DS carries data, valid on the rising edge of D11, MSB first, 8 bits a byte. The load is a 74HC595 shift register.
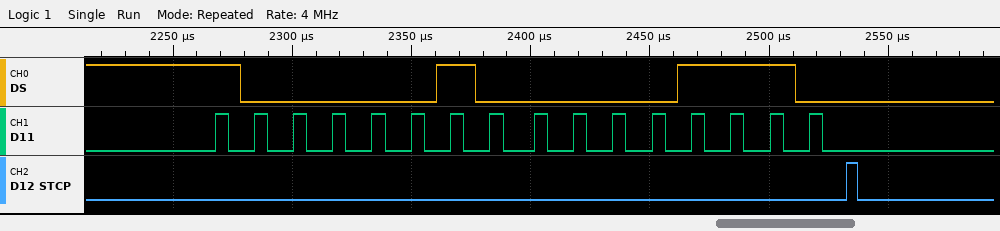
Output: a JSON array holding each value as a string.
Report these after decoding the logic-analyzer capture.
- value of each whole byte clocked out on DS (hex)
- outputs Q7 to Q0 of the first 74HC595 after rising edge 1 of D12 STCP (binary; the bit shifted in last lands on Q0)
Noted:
["0x82 0x0E", "00001110"]
